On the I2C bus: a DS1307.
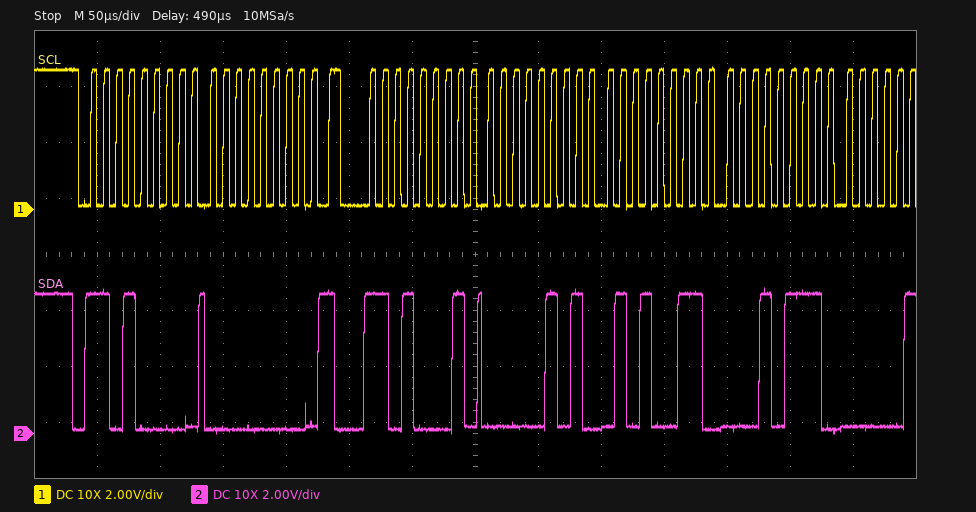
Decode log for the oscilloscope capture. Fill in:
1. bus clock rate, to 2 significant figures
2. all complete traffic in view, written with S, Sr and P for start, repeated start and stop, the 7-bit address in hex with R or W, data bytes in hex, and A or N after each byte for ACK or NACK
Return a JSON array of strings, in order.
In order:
["100 kHz", "S 68W A 00 A Sr 68R A 05 A 53 A 17 A"]
